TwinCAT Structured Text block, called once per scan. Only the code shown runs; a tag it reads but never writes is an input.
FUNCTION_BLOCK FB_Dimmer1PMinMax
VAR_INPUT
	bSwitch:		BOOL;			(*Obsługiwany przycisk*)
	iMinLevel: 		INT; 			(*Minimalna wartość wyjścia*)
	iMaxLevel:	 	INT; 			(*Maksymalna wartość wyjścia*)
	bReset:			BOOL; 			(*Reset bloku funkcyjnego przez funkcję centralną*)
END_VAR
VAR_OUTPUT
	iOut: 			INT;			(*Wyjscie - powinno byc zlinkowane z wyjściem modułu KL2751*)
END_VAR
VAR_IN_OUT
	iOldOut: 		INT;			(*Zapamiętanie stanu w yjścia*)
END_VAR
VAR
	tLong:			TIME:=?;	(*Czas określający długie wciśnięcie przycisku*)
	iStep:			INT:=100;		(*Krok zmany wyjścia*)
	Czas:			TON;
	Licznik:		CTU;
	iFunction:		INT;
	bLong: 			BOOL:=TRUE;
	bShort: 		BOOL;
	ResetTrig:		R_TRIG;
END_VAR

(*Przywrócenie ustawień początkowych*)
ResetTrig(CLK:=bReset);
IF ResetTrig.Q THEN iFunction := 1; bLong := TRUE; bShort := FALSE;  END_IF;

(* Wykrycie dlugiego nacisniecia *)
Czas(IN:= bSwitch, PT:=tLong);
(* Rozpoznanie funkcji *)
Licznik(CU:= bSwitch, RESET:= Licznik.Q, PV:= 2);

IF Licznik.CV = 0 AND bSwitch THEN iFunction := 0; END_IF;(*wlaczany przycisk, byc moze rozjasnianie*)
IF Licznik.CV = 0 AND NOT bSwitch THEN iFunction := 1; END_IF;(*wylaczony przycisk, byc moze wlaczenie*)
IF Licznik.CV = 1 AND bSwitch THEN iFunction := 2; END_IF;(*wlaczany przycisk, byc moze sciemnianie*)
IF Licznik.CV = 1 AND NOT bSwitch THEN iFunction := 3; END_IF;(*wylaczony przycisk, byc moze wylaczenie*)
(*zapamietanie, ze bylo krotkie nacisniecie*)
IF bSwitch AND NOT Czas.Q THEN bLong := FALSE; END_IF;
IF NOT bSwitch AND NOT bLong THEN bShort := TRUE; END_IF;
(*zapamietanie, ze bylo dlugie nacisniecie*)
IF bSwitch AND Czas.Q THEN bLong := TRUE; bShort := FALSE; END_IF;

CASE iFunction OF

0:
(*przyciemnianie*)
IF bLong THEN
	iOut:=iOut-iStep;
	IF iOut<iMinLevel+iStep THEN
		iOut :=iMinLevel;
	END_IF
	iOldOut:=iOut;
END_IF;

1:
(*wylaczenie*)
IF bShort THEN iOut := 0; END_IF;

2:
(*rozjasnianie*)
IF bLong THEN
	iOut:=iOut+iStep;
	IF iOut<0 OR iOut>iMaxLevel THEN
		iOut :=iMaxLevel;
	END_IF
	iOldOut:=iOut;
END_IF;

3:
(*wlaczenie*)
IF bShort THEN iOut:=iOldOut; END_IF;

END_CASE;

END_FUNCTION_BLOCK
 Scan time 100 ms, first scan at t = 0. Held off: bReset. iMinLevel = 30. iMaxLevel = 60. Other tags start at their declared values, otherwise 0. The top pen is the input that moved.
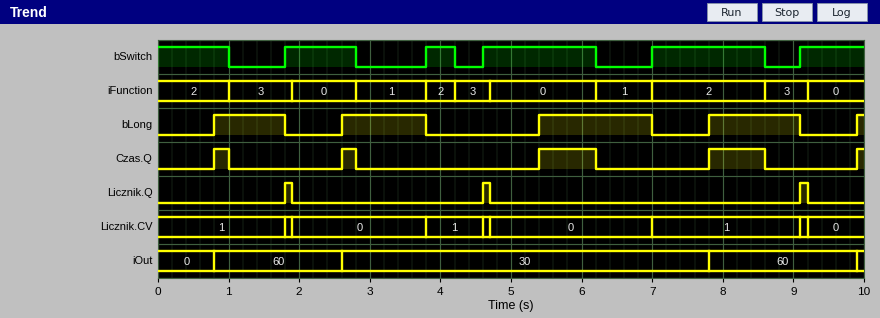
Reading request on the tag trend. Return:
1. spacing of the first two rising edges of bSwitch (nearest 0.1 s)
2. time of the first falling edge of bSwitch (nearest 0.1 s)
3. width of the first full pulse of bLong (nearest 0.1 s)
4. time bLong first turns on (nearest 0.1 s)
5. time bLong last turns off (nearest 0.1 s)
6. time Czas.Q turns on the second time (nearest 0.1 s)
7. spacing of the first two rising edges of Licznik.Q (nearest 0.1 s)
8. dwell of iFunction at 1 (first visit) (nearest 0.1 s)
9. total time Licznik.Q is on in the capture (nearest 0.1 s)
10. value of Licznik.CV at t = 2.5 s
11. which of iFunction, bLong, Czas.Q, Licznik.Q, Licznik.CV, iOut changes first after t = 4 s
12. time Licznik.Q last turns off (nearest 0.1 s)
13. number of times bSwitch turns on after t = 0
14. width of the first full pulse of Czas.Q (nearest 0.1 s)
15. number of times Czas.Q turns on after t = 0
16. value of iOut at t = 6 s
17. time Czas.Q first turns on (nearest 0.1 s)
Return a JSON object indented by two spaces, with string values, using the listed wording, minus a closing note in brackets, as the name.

{
  "spacing of the first two rising edges of bSwitch": "2.0 s",
  "time of the first falling edge of bSwitch": "1.0 s",
  "width of the first full pulse of bLong": "1.0 s",
  "time bLong first turns on": "0.8 s",
  "time bLong last turns off": "9.1 s",
  "time Czas.Q turns on the second time": "2.6 s",
  "spacing of the first two rising edges of Licznik.Q": "2.8 s",
  "dwell of iFunction at 1 (first visit)": "1.0 s",
  "total time Licznik.Q is on in the capture": "0.3 s",
  "value of Licznik.CV at t = 2.5 s": "0",
  "which of iFunction, bLong, Czas.Q, Licznik.Q, Licznik.CV, iOut changes first after t = 4 s": "iFunction",
  "time Licznik.Q last turns off": "9.2 s",
  "number of times bSwitch turns on after t = 0": "5",
  "width of the first full pulse of Czas.Q": "0.2 s",
  "number of times Czas.Q turns on after t = 0": "5",
  "value of iOut at t = 6 s": "30",
  "time Czas.Q first turns on": "0.8 s"
}
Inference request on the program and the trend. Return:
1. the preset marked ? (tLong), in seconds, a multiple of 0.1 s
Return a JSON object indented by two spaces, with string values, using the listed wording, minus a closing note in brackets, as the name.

{
  "the preset marked ? (tLong), in seconds, a multiple of 0.1 s": "0.8 s"
}
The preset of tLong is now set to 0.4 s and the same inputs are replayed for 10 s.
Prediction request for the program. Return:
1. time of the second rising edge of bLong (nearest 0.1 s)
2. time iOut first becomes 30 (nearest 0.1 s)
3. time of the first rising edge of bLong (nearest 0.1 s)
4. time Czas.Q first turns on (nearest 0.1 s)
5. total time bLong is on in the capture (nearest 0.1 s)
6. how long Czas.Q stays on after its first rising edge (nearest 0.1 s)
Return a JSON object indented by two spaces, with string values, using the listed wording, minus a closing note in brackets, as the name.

{
  "time of the second rising edge of bLong": "2.2 s",
  "time iOut first becomes 30": "2.2 s",
  "time of the first rising edge of bLong": "0.4 s",
  "time Czas.Q first turns on": "0.4 s",
  "total time bLong is on in the capture": "7.2 s",
  "how long Czas.Q stays on after its first rising edge": "0.6 s"
}
